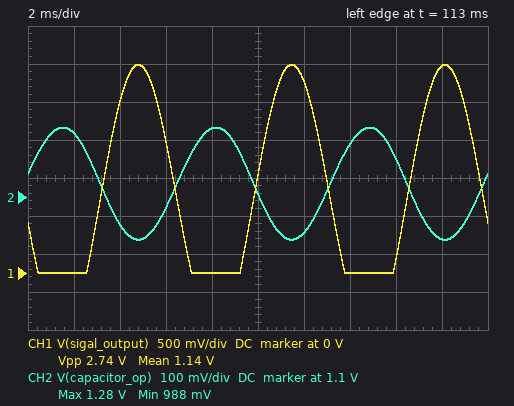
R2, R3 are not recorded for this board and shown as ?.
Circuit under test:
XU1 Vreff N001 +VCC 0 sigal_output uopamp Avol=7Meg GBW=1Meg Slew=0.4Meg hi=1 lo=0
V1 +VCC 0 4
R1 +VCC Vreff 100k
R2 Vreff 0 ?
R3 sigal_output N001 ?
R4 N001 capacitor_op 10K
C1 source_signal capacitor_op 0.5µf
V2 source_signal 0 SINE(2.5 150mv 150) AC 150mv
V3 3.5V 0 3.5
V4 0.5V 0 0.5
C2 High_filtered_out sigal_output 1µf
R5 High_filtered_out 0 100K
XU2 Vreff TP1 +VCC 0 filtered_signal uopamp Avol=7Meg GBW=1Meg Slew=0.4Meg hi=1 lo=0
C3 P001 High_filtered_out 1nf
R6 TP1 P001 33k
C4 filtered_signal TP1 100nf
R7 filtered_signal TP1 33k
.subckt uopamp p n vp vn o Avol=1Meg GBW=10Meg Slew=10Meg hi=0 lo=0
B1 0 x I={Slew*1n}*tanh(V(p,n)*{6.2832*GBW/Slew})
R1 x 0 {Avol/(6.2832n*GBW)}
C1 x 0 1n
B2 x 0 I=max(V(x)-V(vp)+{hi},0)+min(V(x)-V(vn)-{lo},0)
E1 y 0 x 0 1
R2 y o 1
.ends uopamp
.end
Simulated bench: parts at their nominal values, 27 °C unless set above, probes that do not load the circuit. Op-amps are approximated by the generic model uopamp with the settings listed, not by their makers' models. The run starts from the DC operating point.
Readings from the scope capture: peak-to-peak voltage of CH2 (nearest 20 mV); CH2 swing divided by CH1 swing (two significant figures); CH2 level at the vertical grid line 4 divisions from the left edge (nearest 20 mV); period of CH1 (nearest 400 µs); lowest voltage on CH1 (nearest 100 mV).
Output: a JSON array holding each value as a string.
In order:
["300 mV", "0.11", "1.28 V", "6.8 ms", "0 V"]
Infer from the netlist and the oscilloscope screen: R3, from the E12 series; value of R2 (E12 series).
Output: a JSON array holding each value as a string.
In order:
["120 kΩ", "39 kΩ"]
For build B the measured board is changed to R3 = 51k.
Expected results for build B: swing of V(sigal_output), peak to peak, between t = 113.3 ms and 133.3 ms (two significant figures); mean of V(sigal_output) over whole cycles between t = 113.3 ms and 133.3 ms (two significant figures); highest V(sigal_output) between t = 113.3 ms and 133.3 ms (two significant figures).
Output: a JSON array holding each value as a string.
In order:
["1.5 V", "1.1 V", "1.9 V"]
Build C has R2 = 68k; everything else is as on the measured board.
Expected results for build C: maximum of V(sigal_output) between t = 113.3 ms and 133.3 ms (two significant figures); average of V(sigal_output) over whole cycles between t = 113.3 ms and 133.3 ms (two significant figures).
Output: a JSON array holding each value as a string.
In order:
["3.0 V", "1.6 V"]
